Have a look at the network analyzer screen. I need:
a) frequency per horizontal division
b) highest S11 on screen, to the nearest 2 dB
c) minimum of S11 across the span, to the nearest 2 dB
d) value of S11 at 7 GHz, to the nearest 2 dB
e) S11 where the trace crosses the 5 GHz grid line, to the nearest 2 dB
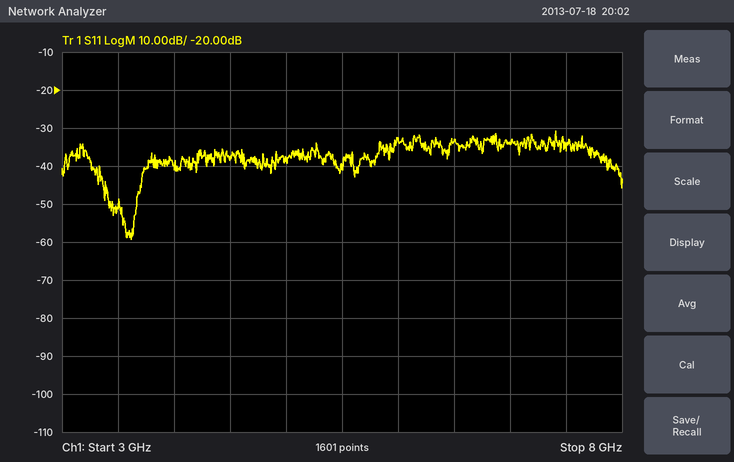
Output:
500 MHz
-30 dB
-60 dB
-34 dB
-38 dB
